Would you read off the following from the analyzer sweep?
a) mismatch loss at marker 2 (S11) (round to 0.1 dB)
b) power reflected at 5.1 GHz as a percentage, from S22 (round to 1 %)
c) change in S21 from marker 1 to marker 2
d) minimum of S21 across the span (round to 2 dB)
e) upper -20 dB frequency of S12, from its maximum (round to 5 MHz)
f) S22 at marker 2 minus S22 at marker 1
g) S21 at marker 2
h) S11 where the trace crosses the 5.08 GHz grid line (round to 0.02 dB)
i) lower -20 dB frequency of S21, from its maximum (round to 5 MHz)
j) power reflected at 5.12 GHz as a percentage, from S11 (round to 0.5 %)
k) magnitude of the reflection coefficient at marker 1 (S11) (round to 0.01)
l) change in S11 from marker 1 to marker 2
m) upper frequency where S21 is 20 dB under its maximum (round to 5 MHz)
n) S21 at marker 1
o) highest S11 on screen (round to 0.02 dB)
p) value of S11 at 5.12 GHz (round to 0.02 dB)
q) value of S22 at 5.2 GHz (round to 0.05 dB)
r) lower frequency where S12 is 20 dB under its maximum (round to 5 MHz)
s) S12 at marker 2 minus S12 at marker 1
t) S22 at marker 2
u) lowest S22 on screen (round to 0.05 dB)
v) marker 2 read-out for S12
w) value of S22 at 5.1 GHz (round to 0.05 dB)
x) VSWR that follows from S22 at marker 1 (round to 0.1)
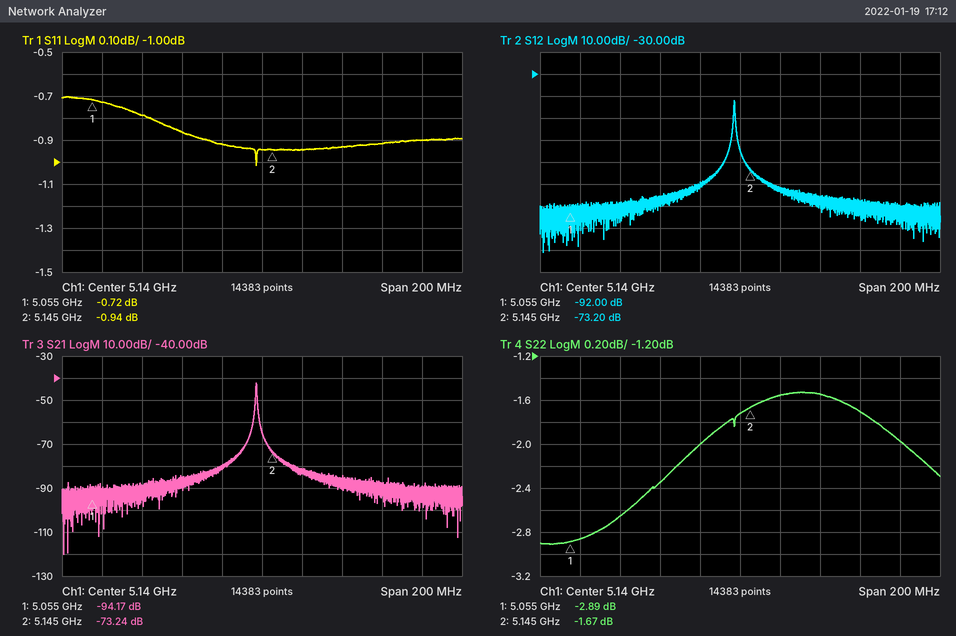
7.1 dB
58 %
20.93 dB
-120 dB
5.140 GHz
1.22 dB
-73.24 dB
-0.78 dB
5.135 GHz
81.0 %
0.92
-0.22 dB
5.140 GHz
-94.17 dB
-0.70 dB
-0.92 dB
-1.70 dB
5.135 GHz
18.80 dB
-1.67 dB
-2.90 dB
-73.20 dB
-2.35 dB
6.1
